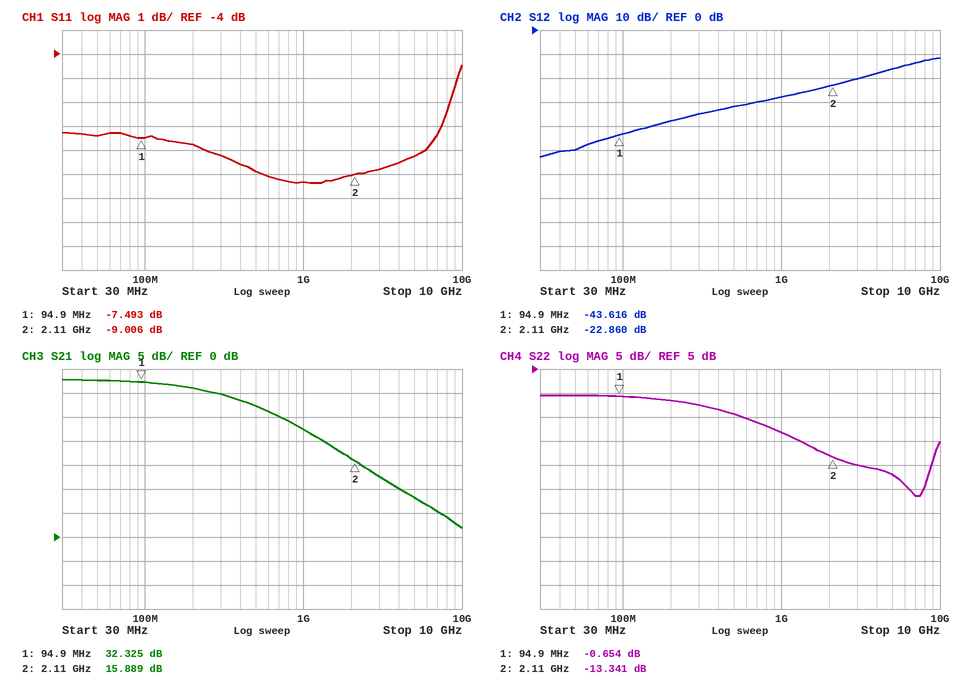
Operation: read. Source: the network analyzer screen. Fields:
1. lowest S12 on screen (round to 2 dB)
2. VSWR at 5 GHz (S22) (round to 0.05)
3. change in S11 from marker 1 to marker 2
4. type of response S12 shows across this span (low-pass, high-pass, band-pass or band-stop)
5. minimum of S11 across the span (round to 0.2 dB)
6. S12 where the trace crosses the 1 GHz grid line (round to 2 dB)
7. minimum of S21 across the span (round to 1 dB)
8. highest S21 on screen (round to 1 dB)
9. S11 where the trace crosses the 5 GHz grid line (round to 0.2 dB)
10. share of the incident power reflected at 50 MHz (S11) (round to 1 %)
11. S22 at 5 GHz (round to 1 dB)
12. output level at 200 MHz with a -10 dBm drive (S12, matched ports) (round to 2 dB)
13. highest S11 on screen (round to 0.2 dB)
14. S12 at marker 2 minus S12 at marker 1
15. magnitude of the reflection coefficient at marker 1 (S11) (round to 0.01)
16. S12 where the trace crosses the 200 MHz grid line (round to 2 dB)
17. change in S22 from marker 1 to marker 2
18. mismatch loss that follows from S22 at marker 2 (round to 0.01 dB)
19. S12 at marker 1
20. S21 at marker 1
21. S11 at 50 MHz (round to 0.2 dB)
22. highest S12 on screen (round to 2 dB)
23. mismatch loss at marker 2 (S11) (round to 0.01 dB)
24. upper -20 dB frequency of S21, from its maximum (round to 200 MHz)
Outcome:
-52 dB
1.35
-1.513 dB
high-pass
-9.4 dB
-28 dB
2 dB
33 dB
-8.2 dB
18 %
-17 dB
-48 dBm
-4.4 dB
20.756 dB
0.42
-38 dB
-12.687 dB
0.21 dB
-43.616 dB
32.325 dB
-7.4 dB
-12 dB
0.58 dB
3.0 GHz
